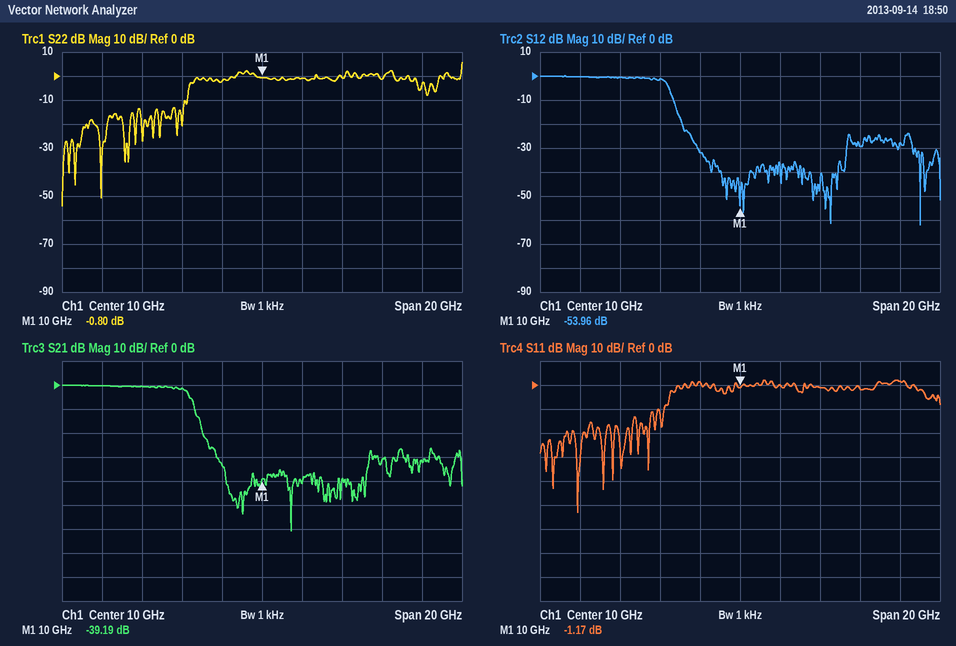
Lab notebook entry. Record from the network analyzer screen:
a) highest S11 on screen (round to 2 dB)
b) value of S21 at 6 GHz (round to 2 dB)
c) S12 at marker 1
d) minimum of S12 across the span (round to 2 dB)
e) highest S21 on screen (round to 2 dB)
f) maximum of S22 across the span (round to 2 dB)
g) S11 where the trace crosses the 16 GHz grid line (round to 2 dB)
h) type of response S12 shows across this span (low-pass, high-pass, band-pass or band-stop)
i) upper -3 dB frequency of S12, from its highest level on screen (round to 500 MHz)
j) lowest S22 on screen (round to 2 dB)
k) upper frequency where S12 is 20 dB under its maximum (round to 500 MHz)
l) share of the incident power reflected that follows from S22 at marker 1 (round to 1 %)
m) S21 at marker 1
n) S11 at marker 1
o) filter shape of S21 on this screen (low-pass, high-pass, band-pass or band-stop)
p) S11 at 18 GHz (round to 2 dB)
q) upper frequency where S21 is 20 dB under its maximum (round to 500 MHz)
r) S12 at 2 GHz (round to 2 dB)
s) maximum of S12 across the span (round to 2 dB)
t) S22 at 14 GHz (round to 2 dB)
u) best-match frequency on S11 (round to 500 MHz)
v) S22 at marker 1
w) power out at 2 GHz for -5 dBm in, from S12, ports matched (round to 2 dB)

2 dB
-2 dB
-53.96 dB
-62 dB
0 dB
6 dB
-2 dB
low-pass
6.5 GHz
-54 dB
7.0 GHz
83 %
-39.19 dB
-1.17 dB
low-pass
2 dB
7.0 GHz
0 dB
0 dB
0 dB
2.0 GHz
-0.80 dB
-6 dBm
